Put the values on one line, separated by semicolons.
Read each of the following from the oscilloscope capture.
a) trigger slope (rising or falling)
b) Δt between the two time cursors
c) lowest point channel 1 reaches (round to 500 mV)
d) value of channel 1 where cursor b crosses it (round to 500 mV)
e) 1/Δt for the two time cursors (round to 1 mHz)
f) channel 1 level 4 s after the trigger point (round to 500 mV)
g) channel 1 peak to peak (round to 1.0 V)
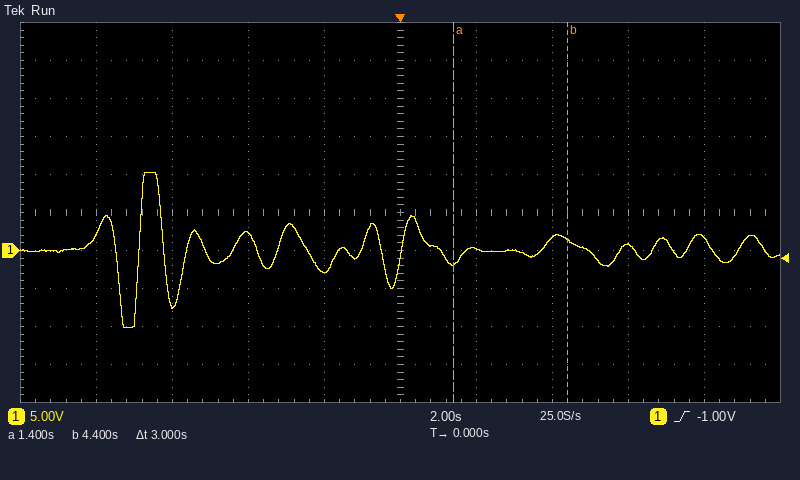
rising; 3 s; -10.0 V; 1.5 V; 333 mHz; 1.5 V; 20.0 V
